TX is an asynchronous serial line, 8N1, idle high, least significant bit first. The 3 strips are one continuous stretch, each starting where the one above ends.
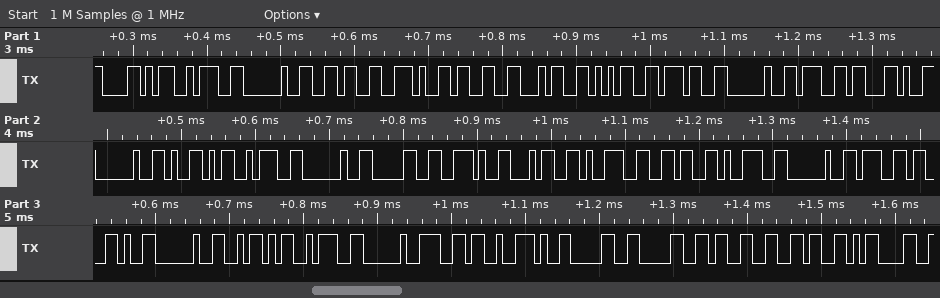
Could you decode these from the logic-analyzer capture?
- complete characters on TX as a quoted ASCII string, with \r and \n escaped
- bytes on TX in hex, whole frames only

"X: 6.3457 g, Y: 0.4969 g, Z: 6.0036\r"
58 3A 20 36 2E 33 34 35 37 20 67 2C 20 59 3A 20 30 2E 34 39 36 39 20 67 2C 20 5A 3A 20 36 2E 30 30 33 36 0D
